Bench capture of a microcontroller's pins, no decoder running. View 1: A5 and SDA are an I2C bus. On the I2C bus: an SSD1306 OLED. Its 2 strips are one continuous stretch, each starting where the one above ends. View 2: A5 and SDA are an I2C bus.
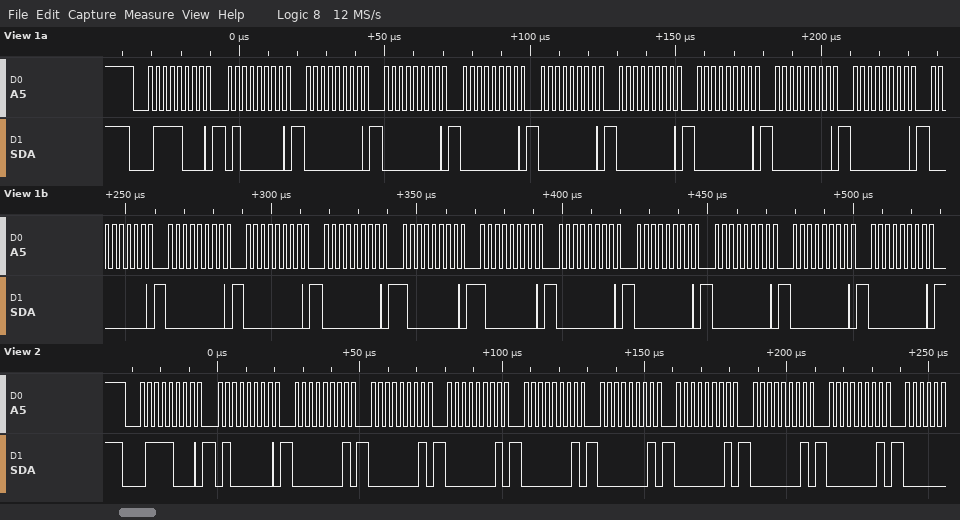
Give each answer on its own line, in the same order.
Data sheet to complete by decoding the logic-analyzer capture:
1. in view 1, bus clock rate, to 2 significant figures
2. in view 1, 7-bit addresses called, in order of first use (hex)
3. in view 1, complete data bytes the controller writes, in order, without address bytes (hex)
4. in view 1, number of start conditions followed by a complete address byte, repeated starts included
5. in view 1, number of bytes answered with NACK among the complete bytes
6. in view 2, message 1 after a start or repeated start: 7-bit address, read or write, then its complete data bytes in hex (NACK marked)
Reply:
400 kHz
0x3C
40 00 00 00 00 00 00 00 00 00 00 00 00 80 80 00 00 00 00 00
1
0
0x3C write: 40 01 01 01 01 01 01 01 01
